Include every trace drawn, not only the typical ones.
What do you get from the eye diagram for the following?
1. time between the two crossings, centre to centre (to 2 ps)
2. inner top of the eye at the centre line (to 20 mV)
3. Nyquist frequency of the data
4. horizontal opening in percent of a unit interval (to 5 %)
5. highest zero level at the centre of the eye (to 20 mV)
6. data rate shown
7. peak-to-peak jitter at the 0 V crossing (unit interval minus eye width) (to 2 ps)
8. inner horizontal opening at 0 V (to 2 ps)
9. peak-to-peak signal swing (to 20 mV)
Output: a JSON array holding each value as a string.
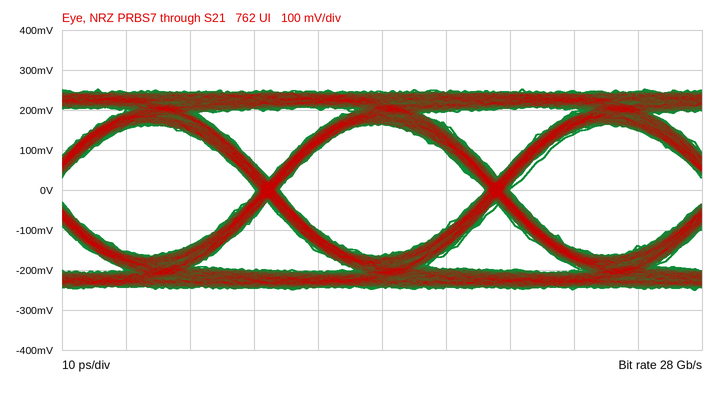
["36 ps", "160 mV", "14 GHz", "90 %", "-160 mV", "28 Gb/s", "4 ps", "32 ps", "500 mV"]
